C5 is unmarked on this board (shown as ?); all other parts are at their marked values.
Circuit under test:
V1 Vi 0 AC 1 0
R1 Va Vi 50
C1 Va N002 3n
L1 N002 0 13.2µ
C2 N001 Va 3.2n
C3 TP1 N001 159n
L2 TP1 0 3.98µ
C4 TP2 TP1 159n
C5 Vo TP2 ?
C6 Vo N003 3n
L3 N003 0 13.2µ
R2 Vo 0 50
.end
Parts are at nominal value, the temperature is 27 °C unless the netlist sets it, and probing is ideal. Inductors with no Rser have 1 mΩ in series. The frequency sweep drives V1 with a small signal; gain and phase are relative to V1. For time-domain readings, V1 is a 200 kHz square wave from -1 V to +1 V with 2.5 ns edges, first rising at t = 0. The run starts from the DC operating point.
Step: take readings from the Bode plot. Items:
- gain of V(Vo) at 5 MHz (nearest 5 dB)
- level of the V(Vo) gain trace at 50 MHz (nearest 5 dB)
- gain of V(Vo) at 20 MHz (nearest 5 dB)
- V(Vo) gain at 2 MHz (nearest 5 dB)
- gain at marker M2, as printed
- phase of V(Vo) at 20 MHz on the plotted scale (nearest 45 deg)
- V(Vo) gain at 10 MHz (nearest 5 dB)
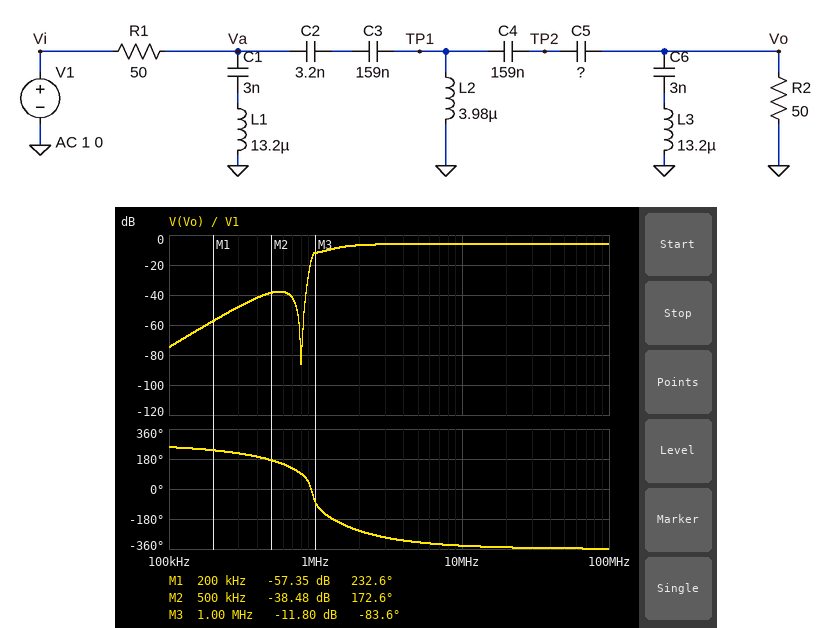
-5 dB
-5 dB
-5 dB
-5 dB
-38.48 dB
-360 deg
-5 dB
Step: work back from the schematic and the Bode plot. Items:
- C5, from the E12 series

1.2 nF
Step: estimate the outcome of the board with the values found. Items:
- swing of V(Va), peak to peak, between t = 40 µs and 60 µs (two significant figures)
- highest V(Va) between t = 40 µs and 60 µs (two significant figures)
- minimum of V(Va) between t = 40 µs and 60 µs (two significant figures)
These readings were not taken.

2.3 V
1.2 V
-1.2 V
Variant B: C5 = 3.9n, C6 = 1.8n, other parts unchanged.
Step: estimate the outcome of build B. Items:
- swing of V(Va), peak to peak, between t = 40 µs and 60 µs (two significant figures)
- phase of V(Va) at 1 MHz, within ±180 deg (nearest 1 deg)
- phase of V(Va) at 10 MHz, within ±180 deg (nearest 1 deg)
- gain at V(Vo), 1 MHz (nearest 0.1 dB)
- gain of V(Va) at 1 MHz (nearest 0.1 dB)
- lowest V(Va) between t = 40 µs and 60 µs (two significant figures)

2.1 V
71 deg
4 deg
-19.0 dB
-26.8 dB
-1.1 V
